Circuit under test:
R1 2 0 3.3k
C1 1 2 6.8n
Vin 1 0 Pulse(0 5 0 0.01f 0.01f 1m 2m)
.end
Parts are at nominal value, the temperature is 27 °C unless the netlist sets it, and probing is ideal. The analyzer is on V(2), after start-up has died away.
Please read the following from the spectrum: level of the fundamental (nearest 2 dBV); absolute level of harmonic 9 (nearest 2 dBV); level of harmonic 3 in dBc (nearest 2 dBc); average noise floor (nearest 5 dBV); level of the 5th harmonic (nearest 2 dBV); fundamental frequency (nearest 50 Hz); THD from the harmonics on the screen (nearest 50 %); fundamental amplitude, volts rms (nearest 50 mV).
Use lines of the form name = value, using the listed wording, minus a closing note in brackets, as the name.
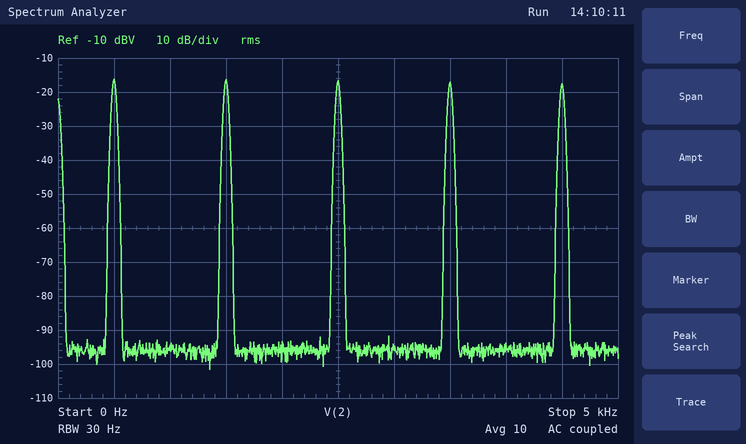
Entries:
level of the fundamental = -16 dBV
absolute level of harmonic 9 = -18 dBV
level of harmonic 3 in dBc = 0 dBc
average noise floor = -95 dBV
level of the 5th harmonic = -16 dBV
fundamental frequency = 500 Hz
THD from the harmonics on the screen = 200 %
fundamental amplitude, volts rms = 150 mV
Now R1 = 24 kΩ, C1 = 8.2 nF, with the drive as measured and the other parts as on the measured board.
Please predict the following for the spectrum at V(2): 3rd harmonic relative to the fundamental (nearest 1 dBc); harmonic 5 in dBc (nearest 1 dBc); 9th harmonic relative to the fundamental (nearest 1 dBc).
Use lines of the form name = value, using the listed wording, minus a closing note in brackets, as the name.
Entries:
3rd harmonic relative to the fundamental = -5 dBc
harmonic 5 in dBc = -9 dBc
9th harmonic relative to the fundamental = -14 dBc
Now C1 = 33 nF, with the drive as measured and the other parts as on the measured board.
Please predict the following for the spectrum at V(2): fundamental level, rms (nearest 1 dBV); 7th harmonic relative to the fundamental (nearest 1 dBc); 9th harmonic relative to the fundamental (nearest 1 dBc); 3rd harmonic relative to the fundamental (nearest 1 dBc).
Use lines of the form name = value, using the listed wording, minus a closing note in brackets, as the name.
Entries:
fundamental level, rms = -3 dBV
7th harmonic relative to the fundamental = -8 dBc
9th harmonic relative to the fundamental = -10 dBc
3rd harmonic relative to the fundamental = -3 dBc
